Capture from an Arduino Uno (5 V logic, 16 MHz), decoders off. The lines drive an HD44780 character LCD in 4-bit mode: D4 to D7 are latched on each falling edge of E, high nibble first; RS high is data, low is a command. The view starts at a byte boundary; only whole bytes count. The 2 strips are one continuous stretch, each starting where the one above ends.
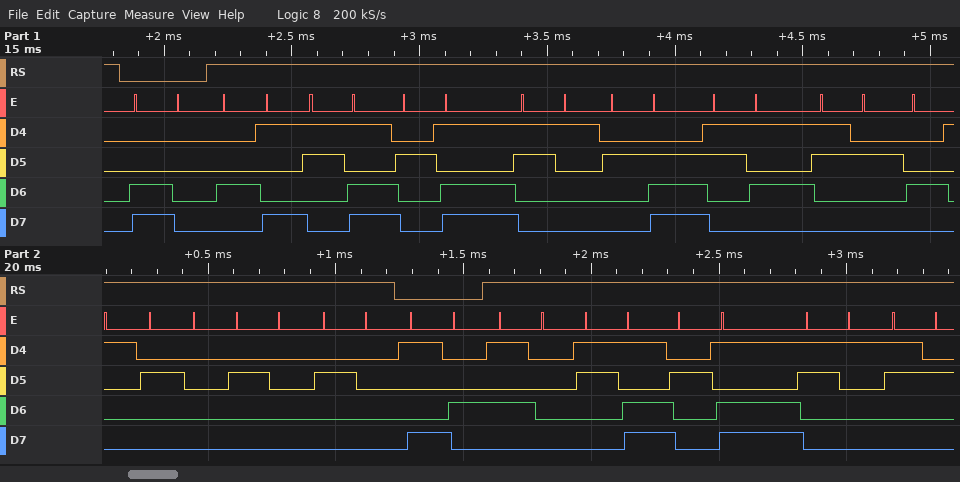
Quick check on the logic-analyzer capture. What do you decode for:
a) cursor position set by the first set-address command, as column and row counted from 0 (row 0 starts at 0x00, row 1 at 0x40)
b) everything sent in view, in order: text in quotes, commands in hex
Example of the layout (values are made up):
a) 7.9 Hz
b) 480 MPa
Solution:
a) column 0, row 1
b) 0xC0 "I=-1.52A   " 0x94 "P=-12"
